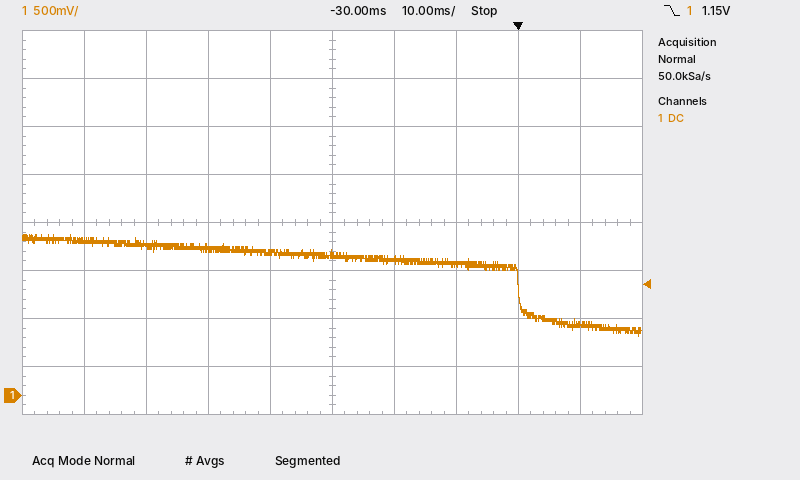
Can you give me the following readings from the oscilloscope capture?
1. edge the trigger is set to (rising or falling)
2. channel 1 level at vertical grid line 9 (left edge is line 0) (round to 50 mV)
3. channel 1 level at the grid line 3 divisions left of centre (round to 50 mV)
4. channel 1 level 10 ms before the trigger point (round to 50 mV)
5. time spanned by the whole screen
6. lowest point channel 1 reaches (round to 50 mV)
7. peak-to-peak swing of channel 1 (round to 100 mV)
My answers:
falling
750 mV
1.55 V
1.35 V
100 ms
600 mV
1.10 V
